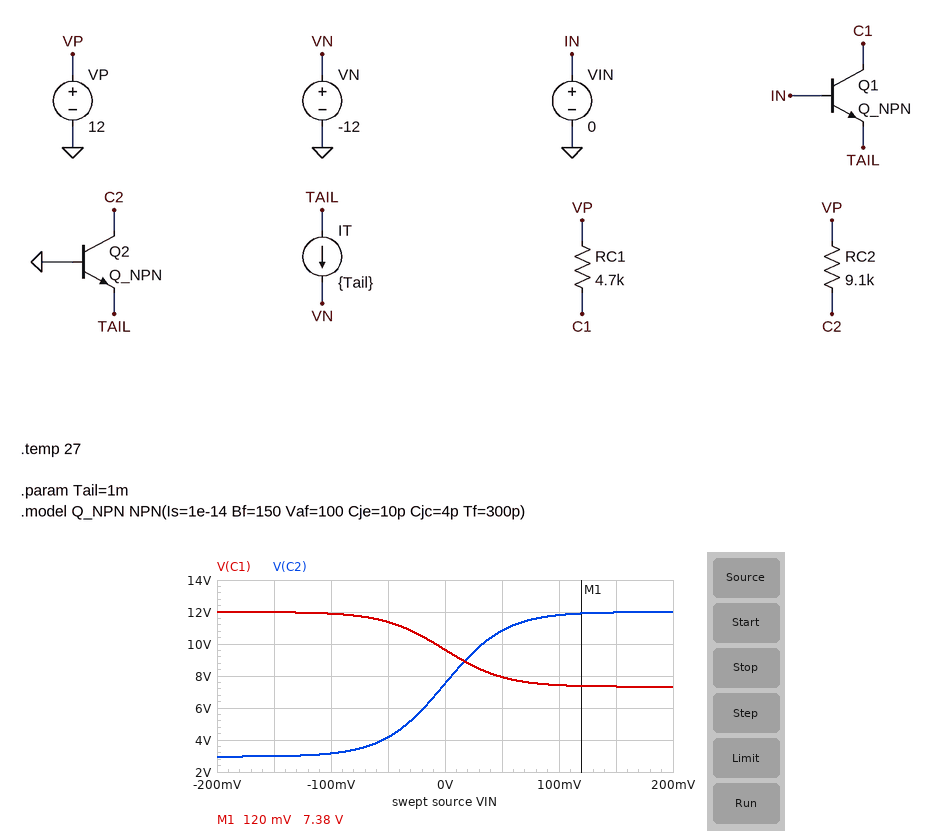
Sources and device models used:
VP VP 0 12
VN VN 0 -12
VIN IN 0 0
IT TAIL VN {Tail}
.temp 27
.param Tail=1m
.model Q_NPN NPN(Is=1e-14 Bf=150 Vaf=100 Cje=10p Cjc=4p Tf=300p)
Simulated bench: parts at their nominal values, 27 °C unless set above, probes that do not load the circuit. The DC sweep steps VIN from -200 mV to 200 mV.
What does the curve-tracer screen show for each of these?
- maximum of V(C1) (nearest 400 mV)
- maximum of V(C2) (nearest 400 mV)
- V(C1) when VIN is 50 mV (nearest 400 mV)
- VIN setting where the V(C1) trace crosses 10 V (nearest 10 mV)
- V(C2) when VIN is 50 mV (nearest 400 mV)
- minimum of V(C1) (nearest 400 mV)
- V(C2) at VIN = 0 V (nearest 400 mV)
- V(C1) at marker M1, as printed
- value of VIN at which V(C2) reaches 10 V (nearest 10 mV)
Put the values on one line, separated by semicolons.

12.0 V; 12.0 V; 8.0 V; -10 mV; 10.8 V; 7.2 V; 7.6 V; 7.38 V; 30 mV
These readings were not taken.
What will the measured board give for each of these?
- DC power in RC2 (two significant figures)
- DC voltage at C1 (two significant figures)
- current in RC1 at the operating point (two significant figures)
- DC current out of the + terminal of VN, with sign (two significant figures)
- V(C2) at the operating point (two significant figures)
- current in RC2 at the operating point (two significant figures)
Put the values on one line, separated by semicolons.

2.2 mW; 9.6 V; 500 µA; -1.0 mA; 7.5 V; 490 µA
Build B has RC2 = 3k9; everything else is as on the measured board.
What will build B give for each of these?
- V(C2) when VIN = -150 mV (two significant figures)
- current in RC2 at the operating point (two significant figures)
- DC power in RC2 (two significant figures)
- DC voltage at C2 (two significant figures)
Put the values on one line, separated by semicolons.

8.1 V; 500 µA; 970 µW; 10 V
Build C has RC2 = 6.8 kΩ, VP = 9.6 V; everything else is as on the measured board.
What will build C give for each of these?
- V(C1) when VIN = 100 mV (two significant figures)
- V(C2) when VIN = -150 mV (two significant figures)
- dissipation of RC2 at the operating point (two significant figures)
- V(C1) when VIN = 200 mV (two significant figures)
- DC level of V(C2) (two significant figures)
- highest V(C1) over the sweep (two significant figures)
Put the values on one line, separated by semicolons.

5.0 V; 2.9 V; 1.7 mW; 4.9 V; 6.2 V; 9.6 V
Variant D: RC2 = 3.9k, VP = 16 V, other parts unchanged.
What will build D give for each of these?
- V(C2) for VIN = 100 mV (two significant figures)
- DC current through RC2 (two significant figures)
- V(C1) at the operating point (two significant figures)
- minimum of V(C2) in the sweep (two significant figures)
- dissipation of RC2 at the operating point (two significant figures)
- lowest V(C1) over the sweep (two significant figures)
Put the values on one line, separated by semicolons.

16 V; 500 µA; 14 V; 12 V; 970 µW; 11 V
